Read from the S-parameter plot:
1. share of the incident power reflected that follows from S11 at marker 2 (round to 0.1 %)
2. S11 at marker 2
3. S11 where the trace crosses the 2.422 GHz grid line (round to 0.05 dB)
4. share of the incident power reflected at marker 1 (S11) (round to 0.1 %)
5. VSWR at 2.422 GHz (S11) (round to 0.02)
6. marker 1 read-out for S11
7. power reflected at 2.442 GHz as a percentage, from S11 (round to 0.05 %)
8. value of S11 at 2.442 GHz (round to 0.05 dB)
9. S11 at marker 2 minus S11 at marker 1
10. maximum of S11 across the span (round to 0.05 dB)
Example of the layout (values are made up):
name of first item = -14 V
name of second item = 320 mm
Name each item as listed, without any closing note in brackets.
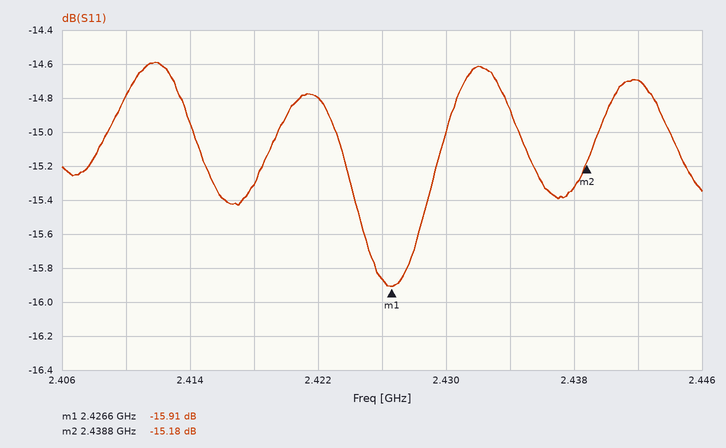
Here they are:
share of the incident power reflected that follows from S11 at marker 2 = 3.0 %
S11 at marker 2 = -15.18 dB
S11 where the trace crosses the 2.422 GHz grid line = -14.80 dB
share of the incident power reflected at marker 1 (S11) = 2.6 %
VSWR at 2.422 GHz (S11) = 1.44
marker 1 read-out for S11 = -15.91 dB
power reflected at 2.442 GHz as a percentage, from S11 = 3.40 %
value of S11 at 2.442 GHz = -14.70 dB
S11 at marker 2 minus S11 at marker 1 = 0.73 dB
maximum of S11 across the span = -14.60 dB
